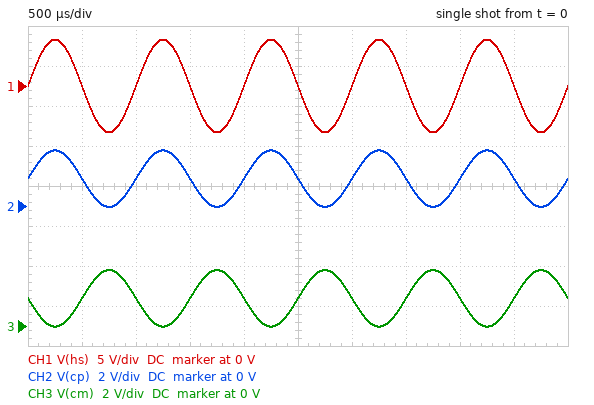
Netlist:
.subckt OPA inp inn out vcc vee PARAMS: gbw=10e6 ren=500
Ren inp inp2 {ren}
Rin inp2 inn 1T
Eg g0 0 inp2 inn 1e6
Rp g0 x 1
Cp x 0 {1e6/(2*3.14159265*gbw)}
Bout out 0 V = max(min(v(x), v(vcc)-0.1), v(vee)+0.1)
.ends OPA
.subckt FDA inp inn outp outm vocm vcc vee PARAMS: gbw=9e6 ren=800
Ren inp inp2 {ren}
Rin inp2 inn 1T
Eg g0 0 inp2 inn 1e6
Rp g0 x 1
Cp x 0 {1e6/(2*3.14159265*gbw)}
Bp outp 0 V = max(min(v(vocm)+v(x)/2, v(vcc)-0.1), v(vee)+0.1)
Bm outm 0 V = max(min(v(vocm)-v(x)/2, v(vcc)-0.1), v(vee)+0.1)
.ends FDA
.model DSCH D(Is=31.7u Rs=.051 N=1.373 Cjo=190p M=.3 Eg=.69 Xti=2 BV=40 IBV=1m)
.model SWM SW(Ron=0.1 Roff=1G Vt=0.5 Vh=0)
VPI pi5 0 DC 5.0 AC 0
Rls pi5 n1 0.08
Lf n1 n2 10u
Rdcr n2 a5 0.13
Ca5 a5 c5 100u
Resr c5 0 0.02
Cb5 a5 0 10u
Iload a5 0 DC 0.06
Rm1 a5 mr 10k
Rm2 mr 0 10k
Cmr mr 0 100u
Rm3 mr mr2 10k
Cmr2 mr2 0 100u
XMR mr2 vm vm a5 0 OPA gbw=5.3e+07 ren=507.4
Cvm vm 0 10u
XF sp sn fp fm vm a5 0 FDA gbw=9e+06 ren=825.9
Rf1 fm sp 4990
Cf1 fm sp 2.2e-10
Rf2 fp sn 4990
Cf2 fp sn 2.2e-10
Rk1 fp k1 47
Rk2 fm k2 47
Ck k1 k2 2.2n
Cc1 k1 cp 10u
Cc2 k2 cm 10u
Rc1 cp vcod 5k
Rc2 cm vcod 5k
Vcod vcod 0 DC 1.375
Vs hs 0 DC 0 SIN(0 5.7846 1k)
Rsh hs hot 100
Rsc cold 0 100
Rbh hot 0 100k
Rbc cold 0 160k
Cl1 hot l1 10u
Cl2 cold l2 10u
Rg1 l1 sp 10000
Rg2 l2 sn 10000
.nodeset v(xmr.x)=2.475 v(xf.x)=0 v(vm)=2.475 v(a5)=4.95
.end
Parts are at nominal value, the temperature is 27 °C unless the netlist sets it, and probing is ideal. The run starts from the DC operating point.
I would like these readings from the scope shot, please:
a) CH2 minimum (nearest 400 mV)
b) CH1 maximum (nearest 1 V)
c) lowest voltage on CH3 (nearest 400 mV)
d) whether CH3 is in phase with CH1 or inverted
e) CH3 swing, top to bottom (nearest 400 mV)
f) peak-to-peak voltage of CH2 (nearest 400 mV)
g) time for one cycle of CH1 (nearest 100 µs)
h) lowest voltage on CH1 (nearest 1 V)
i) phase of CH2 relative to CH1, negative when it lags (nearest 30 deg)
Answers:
0 V
6 V
0 V
inverted
2.8 V
2.8 V
1.0 ms
-6 V
0 deg
